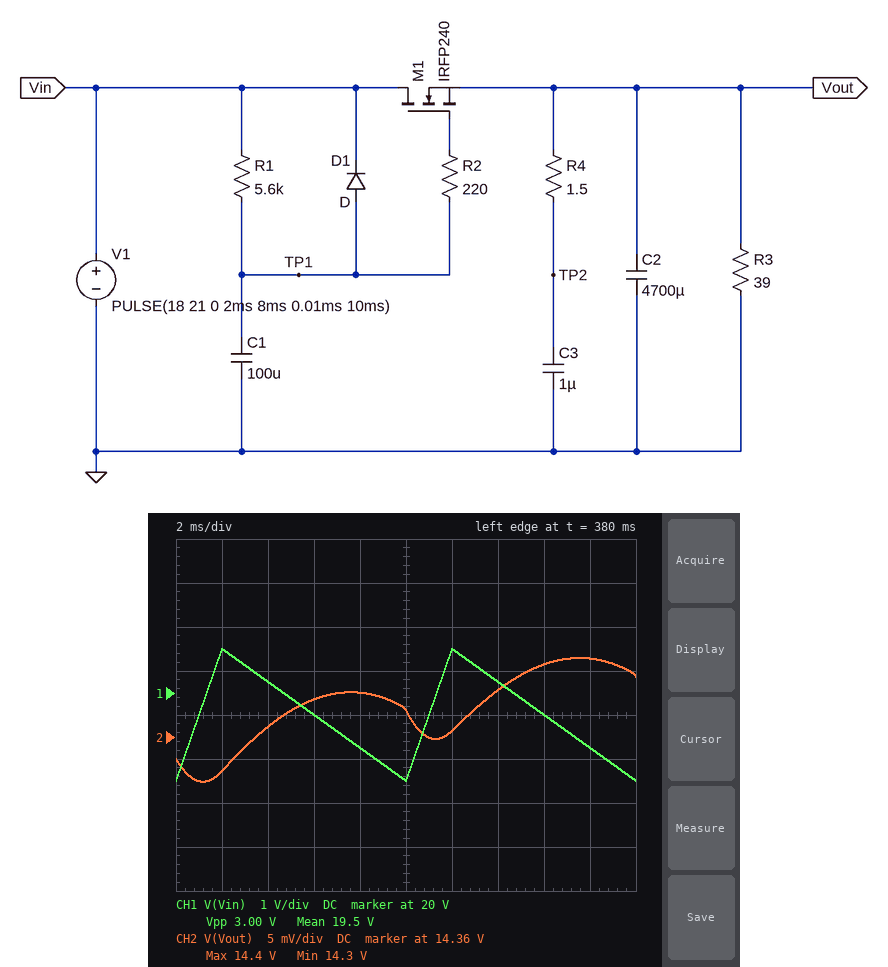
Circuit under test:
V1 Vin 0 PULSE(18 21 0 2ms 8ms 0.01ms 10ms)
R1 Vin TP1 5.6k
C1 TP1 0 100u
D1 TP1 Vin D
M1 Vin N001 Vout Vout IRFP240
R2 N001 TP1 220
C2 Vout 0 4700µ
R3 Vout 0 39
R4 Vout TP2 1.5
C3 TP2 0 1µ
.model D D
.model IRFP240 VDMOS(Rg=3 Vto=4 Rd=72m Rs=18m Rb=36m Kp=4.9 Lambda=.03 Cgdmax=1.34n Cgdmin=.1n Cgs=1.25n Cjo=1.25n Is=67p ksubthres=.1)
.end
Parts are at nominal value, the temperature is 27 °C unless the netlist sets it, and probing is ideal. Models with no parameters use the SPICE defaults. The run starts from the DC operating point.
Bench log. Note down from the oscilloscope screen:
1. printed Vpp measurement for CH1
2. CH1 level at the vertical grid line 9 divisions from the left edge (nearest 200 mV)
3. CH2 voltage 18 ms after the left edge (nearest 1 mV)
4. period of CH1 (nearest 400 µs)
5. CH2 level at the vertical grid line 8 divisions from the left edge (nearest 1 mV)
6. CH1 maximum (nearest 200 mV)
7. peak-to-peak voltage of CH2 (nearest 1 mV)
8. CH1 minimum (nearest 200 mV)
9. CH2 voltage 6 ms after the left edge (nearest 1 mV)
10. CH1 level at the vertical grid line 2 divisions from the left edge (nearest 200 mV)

3.00 V
18.8 V
14.364 V
10.0 ms
14.363 V
21.0 V
14 mV
18.0 V
14.359 V
20.2 V
